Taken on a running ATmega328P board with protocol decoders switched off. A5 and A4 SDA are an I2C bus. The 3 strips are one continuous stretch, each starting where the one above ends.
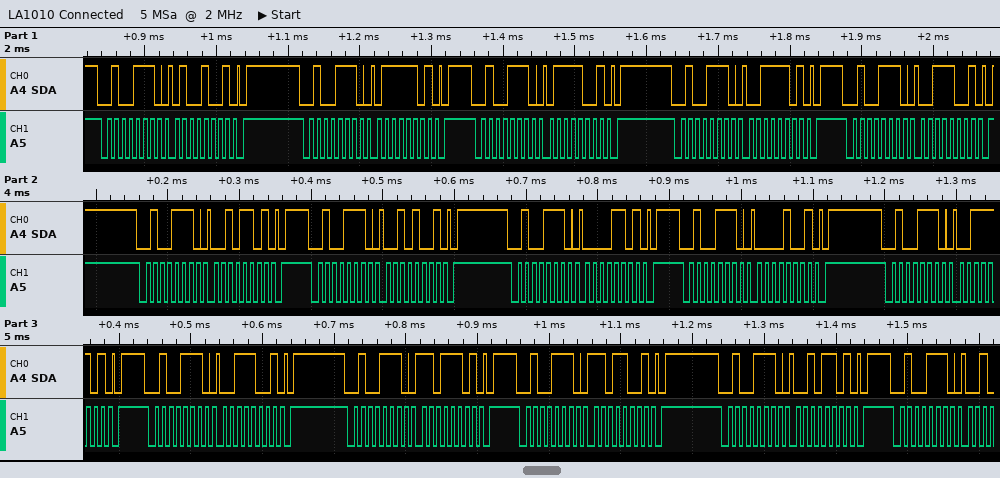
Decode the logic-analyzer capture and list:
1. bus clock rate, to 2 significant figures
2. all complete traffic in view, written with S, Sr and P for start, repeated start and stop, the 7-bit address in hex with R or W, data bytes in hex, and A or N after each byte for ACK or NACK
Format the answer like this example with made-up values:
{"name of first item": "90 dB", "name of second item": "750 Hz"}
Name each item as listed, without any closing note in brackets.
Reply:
{"bus clock rate, to 2 significant figures": "100 kHz", "all complete traffic in view, written with S, Sr and P for start, repeated start and stop, the 7-bit address in hex with R or W, data bytes in hex, and A or N after each byte for ACK or NACK": "S 27W A 49 A P S 27W A 7D A P S 27W A 79 A P S 27W A 3D A P S 27W A 39 A P S 27W A 2D A P S 27W A 29 A P S 27W A 0D A P S 27W A 09 A P S 27W A 3D A P S 27W A 39 A P S 27W A DD A P S 27W A D9 A P S 27W A 2D A P S 27W A"}
